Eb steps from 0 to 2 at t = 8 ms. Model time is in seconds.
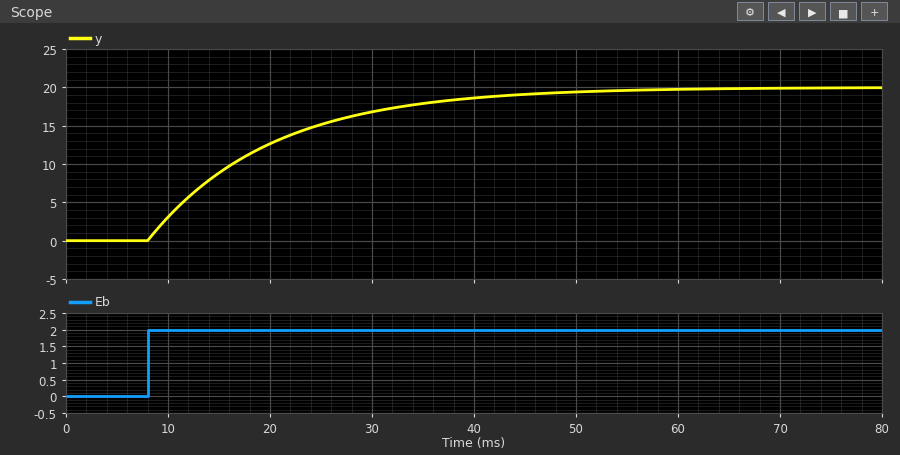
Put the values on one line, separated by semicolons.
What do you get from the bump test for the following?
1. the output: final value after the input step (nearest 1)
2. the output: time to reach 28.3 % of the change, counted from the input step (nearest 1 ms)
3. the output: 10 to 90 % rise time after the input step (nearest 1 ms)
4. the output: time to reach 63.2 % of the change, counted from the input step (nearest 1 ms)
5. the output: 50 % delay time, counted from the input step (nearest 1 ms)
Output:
20; 4 ms; 26 ms; 12 ms; 8 ms
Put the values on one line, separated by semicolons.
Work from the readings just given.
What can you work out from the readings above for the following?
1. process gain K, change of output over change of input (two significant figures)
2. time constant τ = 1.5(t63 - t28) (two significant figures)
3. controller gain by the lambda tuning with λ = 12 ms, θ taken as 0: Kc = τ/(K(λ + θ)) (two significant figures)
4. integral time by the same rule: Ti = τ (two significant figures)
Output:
10; 12 ms; 0.10; 12 ms
